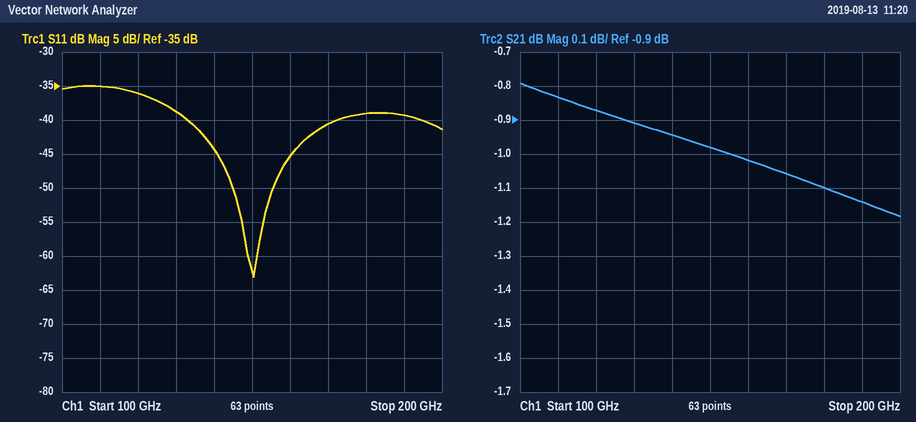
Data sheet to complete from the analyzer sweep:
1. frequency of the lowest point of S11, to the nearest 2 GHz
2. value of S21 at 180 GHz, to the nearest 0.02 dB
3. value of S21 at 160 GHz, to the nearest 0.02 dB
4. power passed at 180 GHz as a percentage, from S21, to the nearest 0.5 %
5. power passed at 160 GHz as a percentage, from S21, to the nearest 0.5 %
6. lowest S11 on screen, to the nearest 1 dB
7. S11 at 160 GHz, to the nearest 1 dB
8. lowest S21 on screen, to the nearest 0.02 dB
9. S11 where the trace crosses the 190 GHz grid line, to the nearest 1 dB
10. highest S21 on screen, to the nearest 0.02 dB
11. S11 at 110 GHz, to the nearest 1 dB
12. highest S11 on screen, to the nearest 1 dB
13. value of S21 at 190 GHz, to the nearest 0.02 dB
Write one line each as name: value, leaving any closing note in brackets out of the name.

frequency of the lowest point of S11, to the nearest 2 GHz: 150 GHz
value of S21 at 180 GHz, to the nearest 0.02 dB: -1.10 dB
value of S21 at 160 GHz, to the nearest 0.02 dB: -1.02 dB
power passed at 180 GHz as a percentage, from S21, to the nearest 0.5 %: 77.5 %
power passed at 160 GHz as a percentage, from S21, to the nearest 0.5 %: 79.0 %
lowest S11 on screen, to the nearest 1 dB: -63 dB
S11 at 160 GHz, to the nearest 1 dB: -45 dB
lowest S21 on screen, to the nearest 0.02 dB: -1.18 dB
S11 where the trace crosses the 190 GHz grid line, to the nearest 1 dB: -39 dB
highest S21 on screen, to the nearest 0.02 dB: -0.80 dB
S11 at 110 GHz, to the nearest 1 dB: -35 dB
highest S11 on screen, to the nearest 1 dB: -35 dB
value of S21 at 190 GHz, to the nearest 0.02 dB: -1.14 dB
